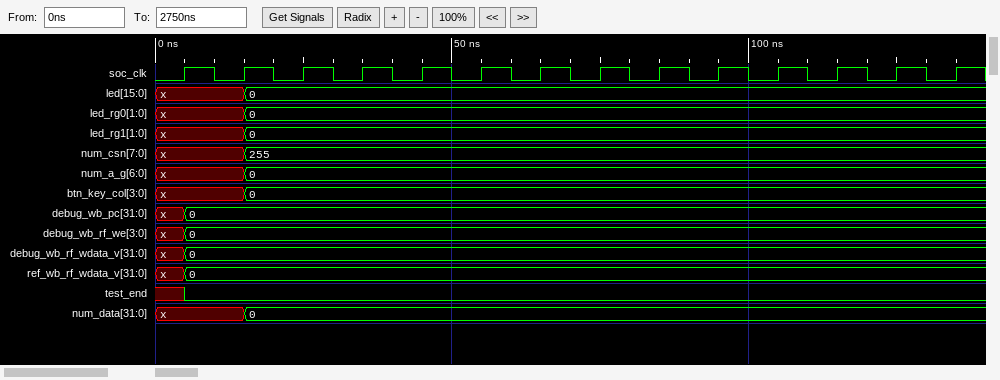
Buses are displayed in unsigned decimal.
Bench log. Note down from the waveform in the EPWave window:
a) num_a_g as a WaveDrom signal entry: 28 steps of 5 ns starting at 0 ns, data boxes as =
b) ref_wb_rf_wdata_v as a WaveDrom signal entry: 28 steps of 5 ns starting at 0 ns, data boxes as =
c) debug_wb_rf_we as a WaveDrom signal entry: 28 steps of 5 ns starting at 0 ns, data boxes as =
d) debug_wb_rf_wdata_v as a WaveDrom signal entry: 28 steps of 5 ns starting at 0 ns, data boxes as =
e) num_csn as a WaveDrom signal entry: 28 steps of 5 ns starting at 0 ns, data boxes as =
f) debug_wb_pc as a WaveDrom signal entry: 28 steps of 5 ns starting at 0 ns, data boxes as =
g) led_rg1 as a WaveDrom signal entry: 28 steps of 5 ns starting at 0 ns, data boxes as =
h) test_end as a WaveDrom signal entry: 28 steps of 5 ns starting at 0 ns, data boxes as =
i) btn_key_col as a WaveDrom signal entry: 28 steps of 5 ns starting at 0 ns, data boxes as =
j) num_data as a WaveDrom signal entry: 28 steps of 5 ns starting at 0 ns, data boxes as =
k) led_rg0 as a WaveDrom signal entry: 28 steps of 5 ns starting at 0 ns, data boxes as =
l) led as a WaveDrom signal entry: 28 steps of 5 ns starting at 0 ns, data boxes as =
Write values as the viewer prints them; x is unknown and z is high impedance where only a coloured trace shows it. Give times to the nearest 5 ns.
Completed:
{name: 'num_a_g', wave: 'x..=........................', data: '0'}
{name: 'ref_wb_rf_wdata_v', wave: 'x=..........................', data: '0'}
{name: 'debug_wb_rf_we', wave: 'x=..........................', data: '0'}
{name: 'debug_wb_rf_wdata_v', wave: 'x=..........................', data: '0'}
{name: 'num_csn', wave: 'x..=........................', data: '255'}
{name: 'debug_wb_pc', wave: 'x=..........................', data: '0'}
{name: 'led_rg1', wave: 'x..=........................', data: '0'}
{name: 'test_end', wave: 'x0..........................'}
{name: 'btn_key_col', wave: 'x..=........................', data: '0'}
{name: 'num_data', wave: 'x..=........................', data: '0'}
{name: 'led_rg0', wave: 'x..=........................', data: '0'}
{name: 'led', wave: 'x..=........................', data: '0'}
